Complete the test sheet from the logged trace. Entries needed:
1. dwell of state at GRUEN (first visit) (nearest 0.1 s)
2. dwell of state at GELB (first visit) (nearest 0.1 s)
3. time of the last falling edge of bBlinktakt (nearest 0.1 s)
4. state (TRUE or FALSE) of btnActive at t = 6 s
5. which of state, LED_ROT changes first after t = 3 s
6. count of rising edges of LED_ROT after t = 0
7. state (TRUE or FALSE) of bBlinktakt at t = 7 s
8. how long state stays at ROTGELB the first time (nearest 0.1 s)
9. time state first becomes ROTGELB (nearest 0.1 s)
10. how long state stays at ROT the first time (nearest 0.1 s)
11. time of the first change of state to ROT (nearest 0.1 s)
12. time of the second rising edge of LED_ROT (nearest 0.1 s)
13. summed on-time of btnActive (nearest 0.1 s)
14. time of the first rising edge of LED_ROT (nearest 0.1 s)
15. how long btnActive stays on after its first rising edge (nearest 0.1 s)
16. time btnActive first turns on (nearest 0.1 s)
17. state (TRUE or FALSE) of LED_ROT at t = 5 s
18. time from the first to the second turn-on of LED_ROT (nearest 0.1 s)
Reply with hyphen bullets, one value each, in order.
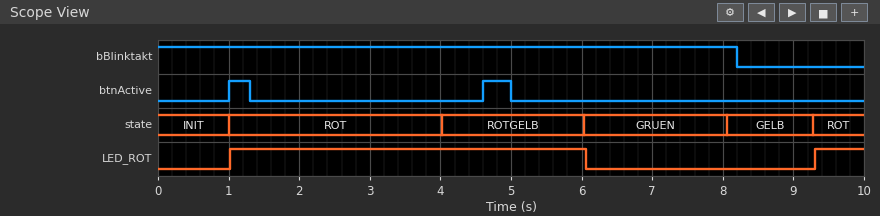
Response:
- 2.0 s
- 1.2 s
- 8.2 s
- FALSE
- state
- 2
- TRUE
- 2.0 s
- 4.0 s
- 3.0 s
- 1.0 s
- 9.3 s
- 0.7 s
- 1.0 s
- 0.3 s
- 1.0 s
- TRUE
- 8.3 s
